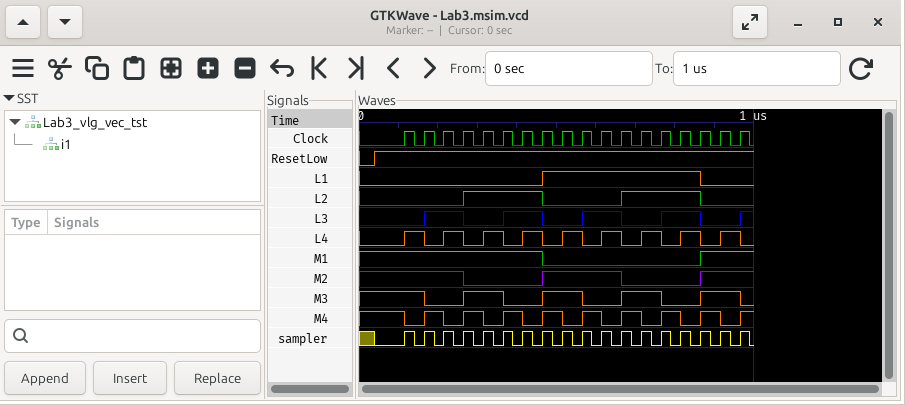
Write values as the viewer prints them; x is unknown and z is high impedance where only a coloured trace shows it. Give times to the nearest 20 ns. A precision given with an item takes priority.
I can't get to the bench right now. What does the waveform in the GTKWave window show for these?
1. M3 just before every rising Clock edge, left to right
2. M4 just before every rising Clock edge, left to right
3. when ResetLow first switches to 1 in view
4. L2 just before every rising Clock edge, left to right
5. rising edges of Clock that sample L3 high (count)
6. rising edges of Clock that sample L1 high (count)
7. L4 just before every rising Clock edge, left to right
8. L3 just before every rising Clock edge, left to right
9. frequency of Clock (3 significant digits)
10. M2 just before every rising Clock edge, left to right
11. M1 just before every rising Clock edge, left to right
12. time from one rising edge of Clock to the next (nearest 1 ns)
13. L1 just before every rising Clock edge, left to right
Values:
1 1 0 0 1 1 0 0 1 1 0 0 1 1 0 0 1 1
1 0 1 0 1 0 1 0 1 0 1 0 1 0 1 0 1 0
40 ns
0 0 0 0 1 1 1 1 0 0 0 0 1 1 1 1 0 0
8
8
0 1 0 1 0 1 0 1 0 1 0 1 0 1 0 1 0 1
0 0 1 1 0 0 1 1 0 0 1 1 0 0 1 1 0 0
20.0 MHz
1 1 1 1 0 0 0 0 1 1 1 1 0 0 0 0 1 1
1 1 1 1 1 1 1 1 0 0 0 0 0 0 0 0 1 1
50 ns
0 0 0 0 0 0 0 0 1 1 1 1 1 1 1 1 0 0
